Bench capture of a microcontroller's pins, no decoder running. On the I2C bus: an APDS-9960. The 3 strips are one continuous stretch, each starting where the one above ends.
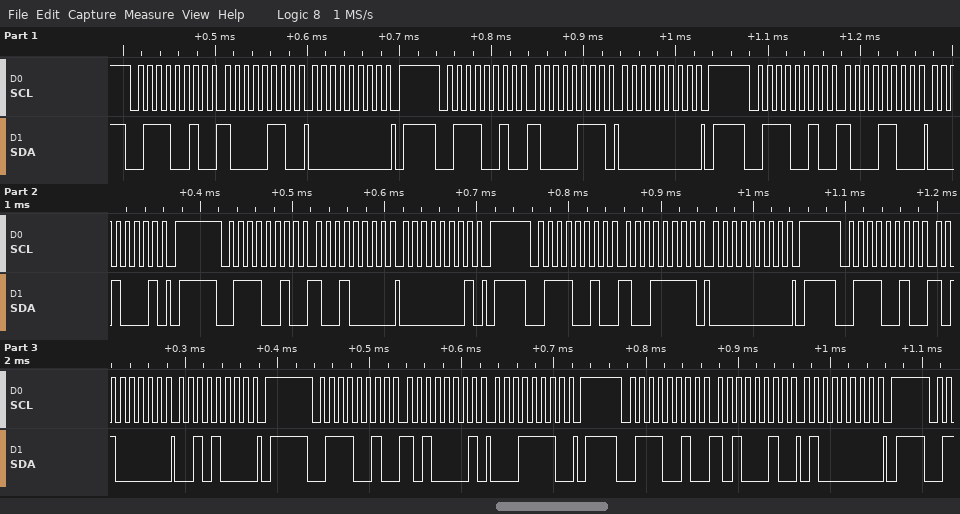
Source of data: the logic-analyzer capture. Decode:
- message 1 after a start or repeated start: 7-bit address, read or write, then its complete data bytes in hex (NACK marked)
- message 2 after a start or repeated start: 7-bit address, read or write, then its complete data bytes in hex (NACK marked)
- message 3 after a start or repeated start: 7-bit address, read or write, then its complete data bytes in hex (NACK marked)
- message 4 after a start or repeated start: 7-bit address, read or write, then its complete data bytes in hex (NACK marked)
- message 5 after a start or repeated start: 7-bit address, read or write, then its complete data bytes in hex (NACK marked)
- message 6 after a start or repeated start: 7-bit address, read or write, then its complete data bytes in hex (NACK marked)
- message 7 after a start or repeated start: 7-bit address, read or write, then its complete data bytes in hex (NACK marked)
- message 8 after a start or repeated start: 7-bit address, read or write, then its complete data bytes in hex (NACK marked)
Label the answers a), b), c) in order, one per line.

a) 0x39 write: 86 00
b) 0x39 write: 87 00
c) 0x39 write: 8C 11
d) 0x39 write: 90 01
e) 0x39 write: 9F 00
f) 0x39 write: A0 28
g) 0x39 write: A1 1E
h) 0x39 write: A2 40
